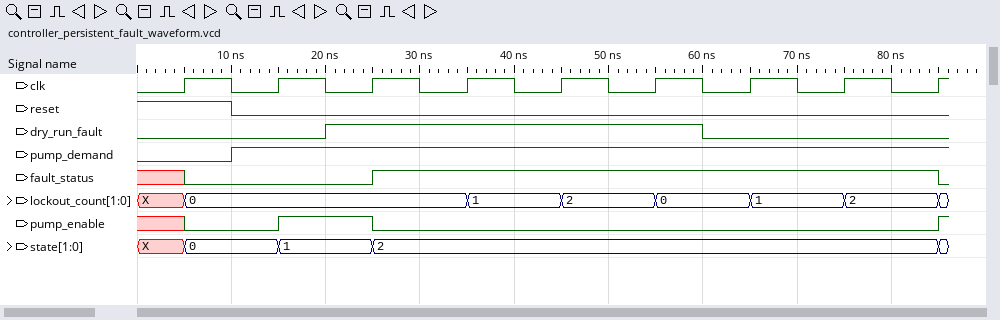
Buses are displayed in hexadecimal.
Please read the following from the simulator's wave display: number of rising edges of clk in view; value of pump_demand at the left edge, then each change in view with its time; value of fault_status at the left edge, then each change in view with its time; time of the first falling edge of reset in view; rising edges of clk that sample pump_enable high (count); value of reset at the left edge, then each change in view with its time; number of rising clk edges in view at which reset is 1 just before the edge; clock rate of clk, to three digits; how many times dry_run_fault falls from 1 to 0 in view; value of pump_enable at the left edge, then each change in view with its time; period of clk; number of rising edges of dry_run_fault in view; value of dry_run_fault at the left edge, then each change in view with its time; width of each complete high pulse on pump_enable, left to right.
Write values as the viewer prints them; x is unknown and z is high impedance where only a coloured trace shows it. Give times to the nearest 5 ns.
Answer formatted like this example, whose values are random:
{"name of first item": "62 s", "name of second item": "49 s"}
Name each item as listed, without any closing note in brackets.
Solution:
{"number of rising edges of clk in view": "9", "value of pump_demand at the left edge, then each change in view with its time": "0, 1 at 10 ns", "value of fault_status at the left edge, then each change in view with its time": "x, 0 at 5 ns, 1 at 25 ns, 0 at 85 ns", "time of the first falling edge of reset in view": "10 ns", "rising edges of clk that sample pump_enable high": "1", "value of reset at the left edge, then each change in view with its time": "1, 0 at 10 ns", "number of rising clk edges in view at which reset is 1 just before the edge": "1", "clock rate of clk, to three digits": "100 MHz", "how many times dry_run_fault falls from 1 to 0 in view": "1", "value of pump_enable at the left edge, then each change in view with its time": "x, 0 at 5 ns, 1 at 15 ns, 0 at 25 ns, 1 at 85 ns", "period of clk": "10 ns", "number of rising edges of dry_run_fault in view": "1", "value of dry_run_fault at the left edge, then each change in view with its time": "0, 1 at 20 ns, 0 at 60 ns", "width of each complete high pulse on pump_enable, left to right": "10 ns"}
